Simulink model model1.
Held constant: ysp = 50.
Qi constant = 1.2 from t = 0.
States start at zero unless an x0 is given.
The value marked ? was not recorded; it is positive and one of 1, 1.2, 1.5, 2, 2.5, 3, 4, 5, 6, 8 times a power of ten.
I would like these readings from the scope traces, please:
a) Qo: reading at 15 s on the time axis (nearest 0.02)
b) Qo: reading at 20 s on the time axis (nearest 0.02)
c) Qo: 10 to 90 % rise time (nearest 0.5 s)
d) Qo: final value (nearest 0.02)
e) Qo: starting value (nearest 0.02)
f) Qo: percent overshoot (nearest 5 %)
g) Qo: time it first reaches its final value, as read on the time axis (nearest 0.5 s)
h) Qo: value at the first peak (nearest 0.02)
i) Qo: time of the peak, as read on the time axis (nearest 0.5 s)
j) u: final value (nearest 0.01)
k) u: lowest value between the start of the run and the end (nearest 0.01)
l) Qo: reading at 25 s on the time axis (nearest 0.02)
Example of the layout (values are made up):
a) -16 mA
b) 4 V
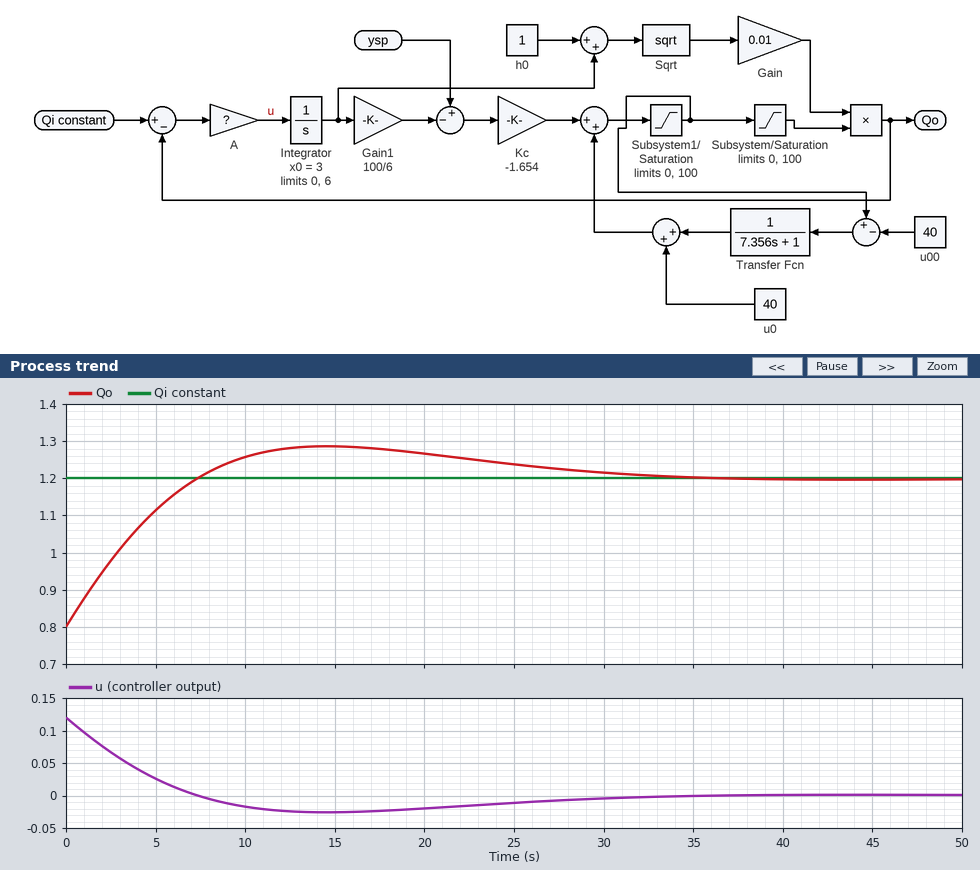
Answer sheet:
a) 1.28
b) 1.26
c) 5.5 s
d) 1.20
e) 0.80
f) 20 %
g) 7.5 s
h) 1.28
i) 14.5 s
j) 0.00
k) -0.03
l) 1.24
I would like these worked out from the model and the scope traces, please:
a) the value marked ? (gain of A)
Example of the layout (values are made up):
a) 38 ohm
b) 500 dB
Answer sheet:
a) 0.3
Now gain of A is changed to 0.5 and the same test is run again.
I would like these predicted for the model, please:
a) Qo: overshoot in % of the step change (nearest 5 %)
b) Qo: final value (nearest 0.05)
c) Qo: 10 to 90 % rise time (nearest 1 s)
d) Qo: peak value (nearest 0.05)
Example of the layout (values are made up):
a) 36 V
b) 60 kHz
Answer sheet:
a) 15 %
b) 1.20
c) 4 s
d) 1.25
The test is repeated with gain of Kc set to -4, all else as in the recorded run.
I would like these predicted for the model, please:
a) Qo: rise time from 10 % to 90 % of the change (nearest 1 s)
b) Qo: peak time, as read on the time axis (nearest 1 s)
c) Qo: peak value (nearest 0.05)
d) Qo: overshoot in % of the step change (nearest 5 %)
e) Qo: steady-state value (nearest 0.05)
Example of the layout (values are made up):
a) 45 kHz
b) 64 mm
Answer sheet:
a) 3 s
b) 9 s
c) 1.25
d) 15 %
e) 1.20
